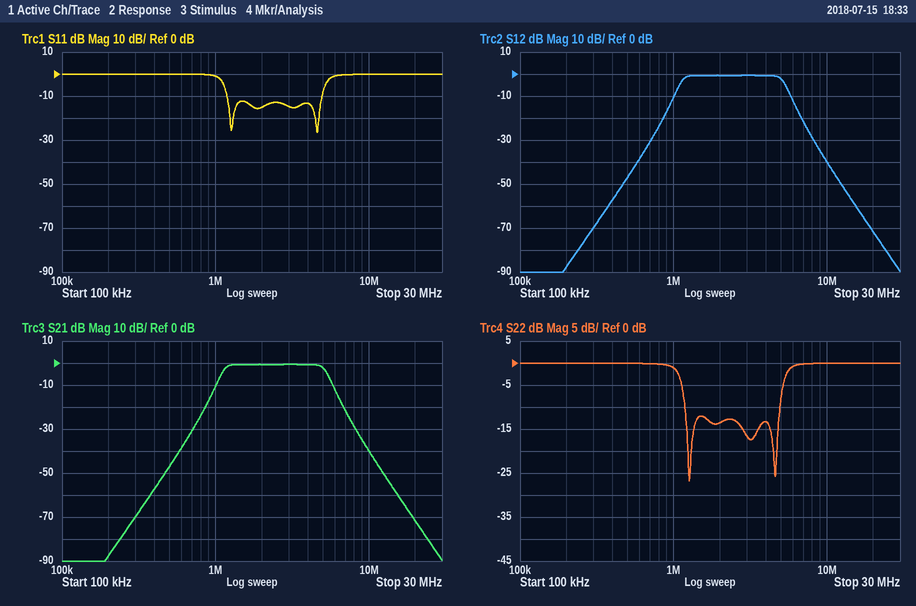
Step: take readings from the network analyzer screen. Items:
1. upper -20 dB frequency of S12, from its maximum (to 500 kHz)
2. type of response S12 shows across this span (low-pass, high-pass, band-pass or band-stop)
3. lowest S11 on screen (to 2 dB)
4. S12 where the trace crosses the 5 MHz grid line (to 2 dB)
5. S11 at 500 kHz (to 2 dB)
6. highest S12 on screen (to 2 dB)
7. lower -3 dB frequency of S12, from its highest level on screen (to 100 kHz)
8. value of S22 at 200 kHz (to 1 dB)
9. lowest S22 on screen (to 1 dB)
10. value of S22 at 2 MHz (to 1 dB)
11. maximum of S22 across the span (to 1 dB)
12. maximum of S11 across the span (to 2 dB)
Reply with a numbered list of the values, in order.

1. 7.0 MHz
2. band-pass
3. -26 dB
4. -2 dB
5. 0 dB
6. 0 dB
7. 1.1 MHz
8. 0 dB
9. -27 dB
10. -14 dB
11. 0 dB
12. 0 dB
